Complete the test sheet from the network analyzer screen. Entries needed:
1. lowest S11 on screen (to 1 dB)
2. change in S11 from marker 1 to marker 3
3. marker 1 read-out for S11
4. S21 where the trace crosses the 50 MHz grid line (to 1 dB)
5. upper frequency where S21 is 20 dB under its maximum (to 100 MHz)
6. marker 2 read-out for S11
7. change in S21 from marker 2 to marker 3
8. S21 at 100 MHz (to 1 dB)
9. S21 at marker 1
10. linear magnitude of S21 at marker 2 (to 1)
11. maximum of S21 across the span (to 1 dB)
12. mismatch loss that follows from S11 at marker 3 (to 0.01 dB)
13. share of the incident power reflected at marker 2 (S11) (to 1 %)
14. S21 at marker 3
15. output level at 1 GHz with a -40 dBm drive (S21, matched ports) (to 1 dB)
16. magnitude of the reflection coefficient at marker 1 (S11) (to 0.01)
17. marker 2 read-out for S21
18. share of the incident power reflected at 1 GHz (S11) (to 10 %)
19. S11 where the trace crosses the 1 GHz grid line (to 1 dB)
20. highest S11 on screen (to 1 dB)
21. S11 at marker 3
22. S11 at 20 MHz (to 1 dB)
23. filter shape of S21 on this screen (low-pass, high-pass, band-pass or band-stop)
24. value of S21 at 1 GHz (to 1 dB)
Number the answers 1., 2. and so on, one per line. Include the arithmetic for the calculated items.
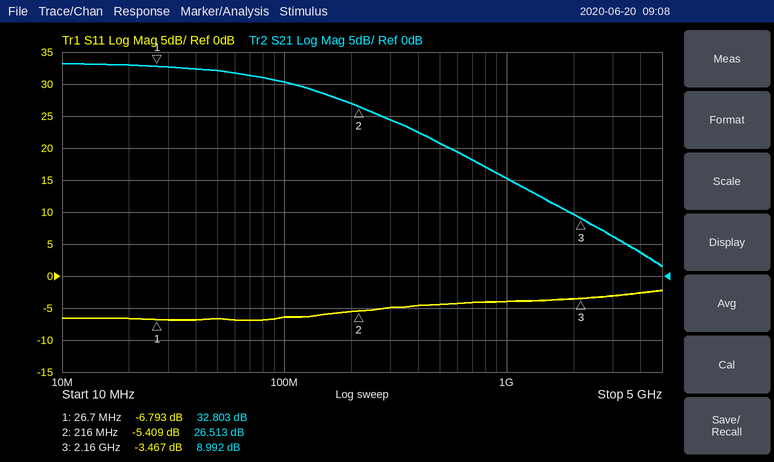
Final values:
1. -7 dB
2. -3.467 − (-6.793) = 3.326 dB
3. -6.793 dB
4. 32 dB
5. 1.3 GHz
6. -5.409 dB
7. 8.992 − (26.513) = -17.521 dB
8. 30 dB
9. 32.803 dB
10. 10^(26.513/20) ≈ 21
11. 33 dB
12. −10 log10(1 − 10^(-3.467/10)) ≈ 2.60 dB
13. 10^(-5.409/10) ≈ 29 %
14. 8.992 dB
15. -40 dBm + (15 dB) = -25 dBm
16. 10^(-6.793/20) ≈ 0.46
17. 26.513 dB
18. 10^(-4/10) ≈ 40 %
19. -4 dB
20. -2 dB
21. -3.467 dB
22. -7 dB
23. low-pass
24. 15 dB
